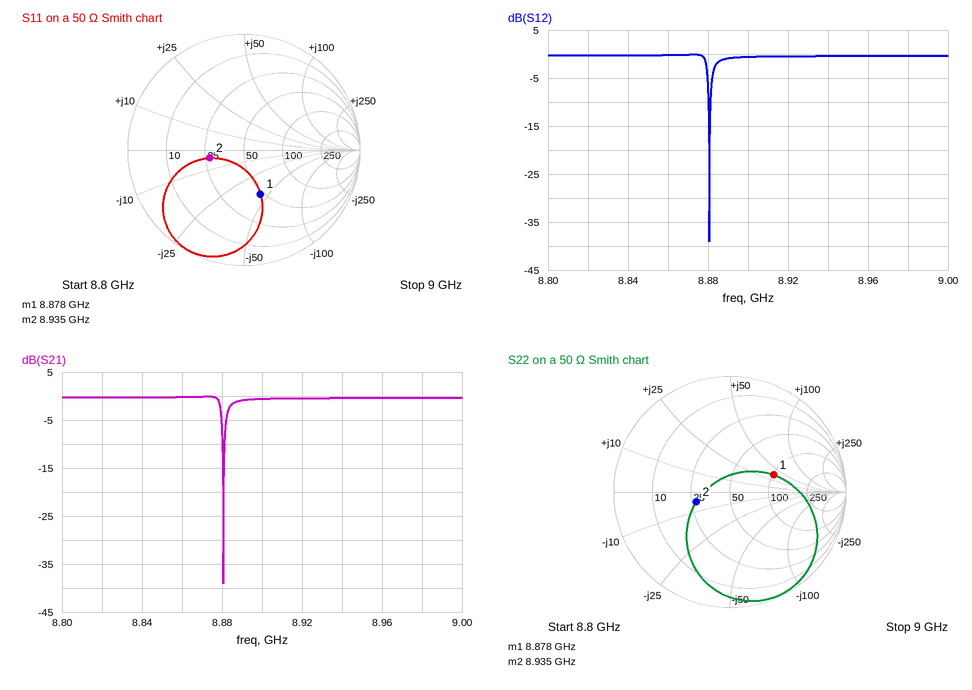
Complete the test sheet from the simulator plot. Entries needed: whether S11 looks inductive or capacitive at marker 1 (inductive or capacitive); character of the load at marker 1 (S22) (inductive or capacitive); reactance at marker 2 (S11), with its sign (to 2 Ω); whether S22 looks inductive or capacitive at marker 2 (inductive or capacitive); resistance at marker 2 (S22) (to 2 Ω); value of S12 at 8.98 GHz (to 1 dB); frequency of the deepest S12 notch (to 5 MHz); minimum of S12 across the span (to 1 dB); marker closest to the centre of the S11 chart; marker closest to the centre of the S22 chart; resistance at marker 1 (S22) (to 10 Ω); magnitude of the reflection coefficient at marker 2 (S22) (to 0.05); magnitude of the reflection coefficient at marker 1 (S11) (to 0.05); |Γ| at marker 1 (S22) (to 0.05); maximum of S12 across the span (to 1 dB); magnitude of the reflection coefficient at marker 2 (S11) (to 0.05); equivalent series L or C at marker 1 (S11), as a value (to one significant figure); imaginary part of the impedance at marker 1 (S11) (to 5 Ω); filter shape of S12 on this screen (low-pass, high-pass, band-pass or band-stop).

capacitive
inductive
-4 Ω
capacitive
28 Ω
0 dB
8.880 GHz
-39 dB
marker 2
marker 2
100 Ω
0.30
0.40
0.40
0 dB
0.30
400 fF
-45 Ω
band-stop
